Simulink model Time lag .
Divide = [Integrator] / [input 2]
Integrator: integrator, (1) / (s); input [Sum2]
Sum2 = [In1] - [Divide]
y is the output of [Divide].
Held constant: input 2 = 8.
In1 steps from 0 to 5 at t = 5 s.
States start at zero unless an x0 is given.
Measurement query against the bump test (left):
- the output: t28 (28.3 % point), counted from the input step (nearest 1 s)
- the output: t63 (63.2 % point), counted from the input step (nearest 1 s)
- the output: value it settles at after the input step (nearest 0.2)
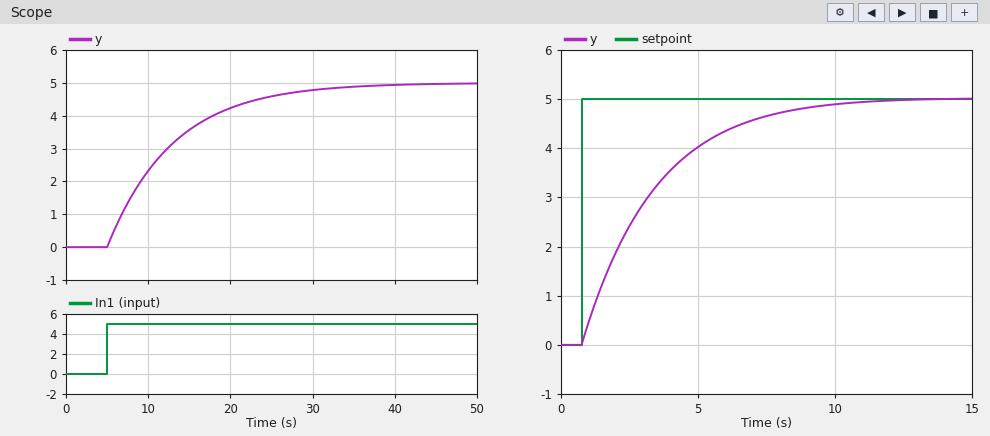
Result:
3 s
8 s
5.0
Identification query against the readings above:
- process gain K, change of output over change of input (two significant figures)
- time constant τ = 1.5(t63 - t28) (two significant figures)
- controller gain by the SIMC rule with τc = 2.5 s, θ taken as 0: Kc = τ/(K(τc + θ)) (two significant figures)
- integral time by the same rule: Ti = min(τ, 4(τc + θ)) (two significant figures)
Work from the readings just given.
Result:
1.0
7.5 s
3.0
7.5 s
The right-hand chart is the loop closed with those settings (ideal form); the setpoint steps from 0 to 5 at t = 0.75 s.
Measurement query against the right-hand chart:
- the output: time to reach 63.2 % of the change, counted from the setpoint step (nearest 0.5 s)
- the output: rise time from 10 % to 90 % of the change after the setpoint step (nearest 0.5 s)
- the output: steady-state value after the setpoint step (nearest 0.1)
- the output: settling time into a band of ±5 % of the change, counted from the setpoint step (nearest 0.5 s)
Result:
2.5 s
5.5 s
5.0
7.5 s
